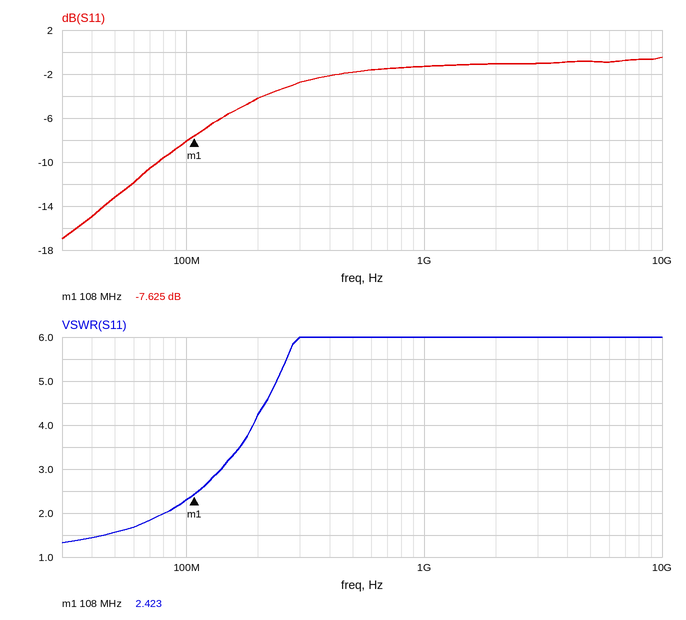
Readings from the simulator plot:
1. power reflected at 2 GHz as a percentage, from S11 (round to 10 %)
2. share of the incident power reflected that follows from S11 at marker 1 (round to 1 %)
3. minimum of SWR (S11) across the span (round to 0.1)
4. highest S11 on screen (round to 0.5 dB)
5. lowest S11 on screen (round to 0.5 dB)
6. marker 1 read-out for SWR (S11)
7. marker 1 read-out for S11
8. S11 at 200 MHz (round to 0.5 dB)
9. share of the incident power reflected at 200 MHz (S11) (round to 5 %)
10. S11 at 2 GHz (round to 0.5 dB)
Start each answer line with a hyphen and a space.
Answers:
- 80 %
- 17 %
- 1.3
- -0.5 dB
- -17.0 dB
- 2.423
- -7.625 dB
- -4.0 dB
- 40 %
- -1.0 dB
